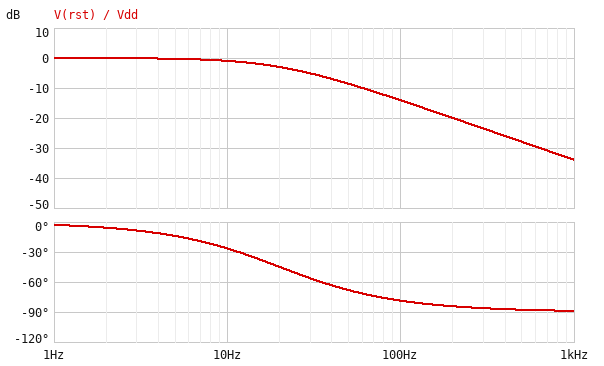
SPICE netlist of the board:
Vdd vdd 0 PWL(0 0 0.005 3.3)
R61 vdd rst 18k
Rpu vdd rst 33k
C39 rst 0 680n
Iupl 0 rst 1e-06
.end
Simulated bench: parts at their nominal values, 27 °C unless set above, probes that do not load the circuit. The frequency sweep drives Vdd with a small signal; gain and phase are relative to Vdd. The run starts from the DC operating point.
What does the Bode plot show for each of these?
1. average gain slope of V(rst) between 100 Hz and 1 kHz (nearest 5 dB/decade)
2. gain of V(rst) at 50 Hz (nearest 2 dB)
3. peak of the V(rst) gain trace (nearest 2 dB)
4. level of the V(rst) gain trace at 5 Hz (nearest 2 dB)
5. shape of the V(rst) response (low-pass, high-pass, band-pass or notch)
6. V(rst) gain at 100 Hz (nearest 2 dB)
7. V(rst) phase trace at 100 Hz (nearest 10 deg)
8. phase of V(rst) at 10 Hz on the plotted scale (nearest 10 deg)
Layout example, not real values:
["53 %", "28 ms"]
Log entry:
["-20 dB/decade", "-8 dB", "0 dB", "0 dB", "low-pass", "-14 dB", "-80 deg", "-30 deg"]
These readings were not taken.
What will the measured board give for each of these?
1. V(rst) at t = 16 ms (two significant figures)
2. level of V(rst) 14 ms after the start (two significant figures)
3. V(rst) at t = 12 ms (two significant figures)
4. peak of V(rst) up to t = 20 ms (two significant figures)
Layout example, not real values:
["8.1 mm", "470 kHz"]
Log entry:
["2.7 V", "2.5 V", "2.3 V", "2.9 V"]
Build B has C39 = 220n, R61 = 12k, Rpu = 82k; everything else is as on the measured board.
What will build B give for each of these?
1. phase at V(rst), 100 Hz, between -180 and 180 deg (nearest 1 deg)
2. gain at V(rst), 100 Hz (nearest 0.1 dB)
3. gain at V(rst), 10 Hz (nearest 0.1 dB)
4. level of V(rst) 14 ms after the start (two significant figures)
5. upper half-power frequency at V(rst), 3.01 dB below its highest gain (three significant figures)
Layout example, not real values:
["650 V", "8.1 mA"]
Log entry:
["-55 deg", "-4.9 dB", "-0.1 dB", "3.3 V", "69.1 Hz"]
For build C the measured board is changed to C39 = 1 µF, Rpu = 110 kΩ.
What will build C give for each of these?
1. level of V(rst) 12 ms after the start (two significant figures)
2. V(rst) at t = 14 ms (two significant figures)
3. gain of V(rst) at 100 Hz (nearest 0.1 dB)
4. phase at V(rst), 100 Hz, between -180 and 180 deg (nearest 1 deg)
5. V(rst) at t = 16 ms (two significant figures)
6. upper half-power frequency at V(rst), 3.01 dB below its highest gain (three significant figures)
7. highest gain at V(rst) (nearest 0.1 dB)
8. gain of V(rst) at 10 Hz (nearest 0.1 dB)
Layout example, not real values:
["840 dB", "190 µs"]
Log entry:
["1.5 V", "1.7 V", "-19.8 dB", "-84 deg", "1.9 V", "10.3 Hz", "0 dB", "-2.9 dB"]
